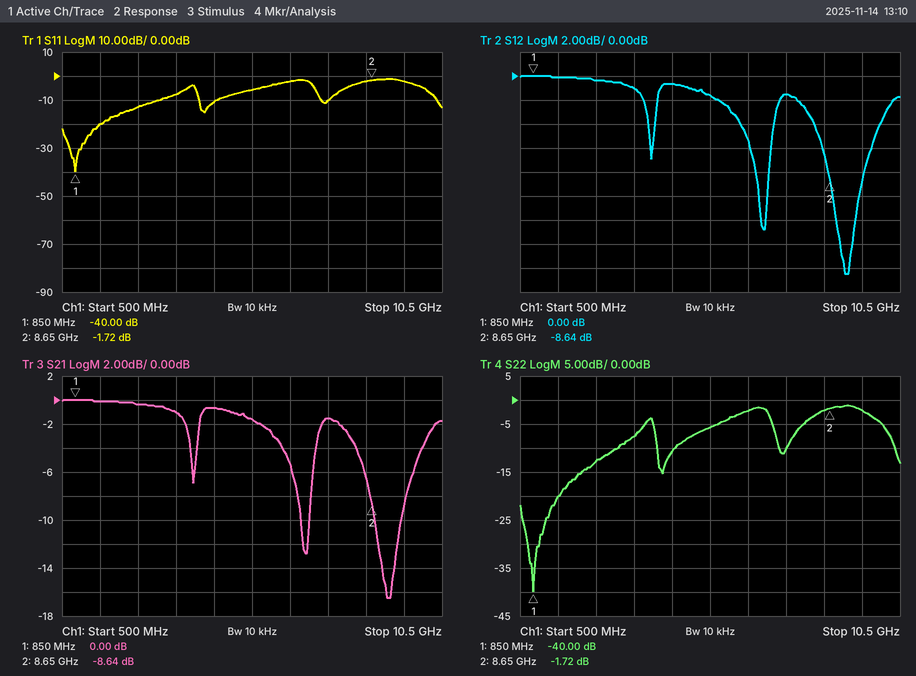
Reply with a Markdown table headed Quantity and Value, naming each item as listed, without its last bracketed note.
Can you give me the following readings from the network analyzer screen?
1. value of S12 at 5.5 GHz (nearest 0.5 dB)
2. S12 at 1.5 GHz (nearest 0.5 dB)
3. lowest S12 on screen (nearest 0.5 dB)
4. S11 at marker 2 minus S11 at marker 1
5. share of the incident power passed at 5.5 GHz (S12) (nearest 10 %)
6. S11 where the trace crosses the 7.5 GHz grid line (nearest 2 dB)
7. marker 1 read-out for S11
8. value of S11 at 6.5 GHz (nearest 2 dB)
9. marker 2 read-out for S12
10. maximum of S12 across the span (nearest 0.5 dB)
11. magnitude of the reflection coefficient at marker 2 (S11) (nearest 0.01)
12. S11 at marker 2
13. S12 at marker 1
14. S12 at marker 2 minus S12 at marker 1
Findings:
| Quantity | Value |
|---|---|
| value of S12 at 5.5 GHz | -1.5 dB |
| S12 at 1.5 GHz | 0.0 dB |
| lowest S12 on screen | -16.5 dB |
| S11 at marker 2 minus S11 at marker 1 | 38.28 dB |
| share of the incident power passed at 5.5 GHz (S12) | 70 % |
| S11 where the trace crosses the 7.5 GHz grid line | -10 dB |
| marker 1 read-out for S11 | -40.00 dB |
| value of S11 at 6.5 GHz | -2 dB |
| marker 2 read-out for S12 | -8.64 dB |
| maximum of S12 across the span | 0.0 dB |
| magnitude of the reflection coefficient at marker 2 (S11) | 0.82 |
| S11 at marker 2 | -1.72 dB |
| S12 at marker 1 | 0.00 dB |
| S12 at marker 2 minus S12 at marker 1 | -8.64 dB |
